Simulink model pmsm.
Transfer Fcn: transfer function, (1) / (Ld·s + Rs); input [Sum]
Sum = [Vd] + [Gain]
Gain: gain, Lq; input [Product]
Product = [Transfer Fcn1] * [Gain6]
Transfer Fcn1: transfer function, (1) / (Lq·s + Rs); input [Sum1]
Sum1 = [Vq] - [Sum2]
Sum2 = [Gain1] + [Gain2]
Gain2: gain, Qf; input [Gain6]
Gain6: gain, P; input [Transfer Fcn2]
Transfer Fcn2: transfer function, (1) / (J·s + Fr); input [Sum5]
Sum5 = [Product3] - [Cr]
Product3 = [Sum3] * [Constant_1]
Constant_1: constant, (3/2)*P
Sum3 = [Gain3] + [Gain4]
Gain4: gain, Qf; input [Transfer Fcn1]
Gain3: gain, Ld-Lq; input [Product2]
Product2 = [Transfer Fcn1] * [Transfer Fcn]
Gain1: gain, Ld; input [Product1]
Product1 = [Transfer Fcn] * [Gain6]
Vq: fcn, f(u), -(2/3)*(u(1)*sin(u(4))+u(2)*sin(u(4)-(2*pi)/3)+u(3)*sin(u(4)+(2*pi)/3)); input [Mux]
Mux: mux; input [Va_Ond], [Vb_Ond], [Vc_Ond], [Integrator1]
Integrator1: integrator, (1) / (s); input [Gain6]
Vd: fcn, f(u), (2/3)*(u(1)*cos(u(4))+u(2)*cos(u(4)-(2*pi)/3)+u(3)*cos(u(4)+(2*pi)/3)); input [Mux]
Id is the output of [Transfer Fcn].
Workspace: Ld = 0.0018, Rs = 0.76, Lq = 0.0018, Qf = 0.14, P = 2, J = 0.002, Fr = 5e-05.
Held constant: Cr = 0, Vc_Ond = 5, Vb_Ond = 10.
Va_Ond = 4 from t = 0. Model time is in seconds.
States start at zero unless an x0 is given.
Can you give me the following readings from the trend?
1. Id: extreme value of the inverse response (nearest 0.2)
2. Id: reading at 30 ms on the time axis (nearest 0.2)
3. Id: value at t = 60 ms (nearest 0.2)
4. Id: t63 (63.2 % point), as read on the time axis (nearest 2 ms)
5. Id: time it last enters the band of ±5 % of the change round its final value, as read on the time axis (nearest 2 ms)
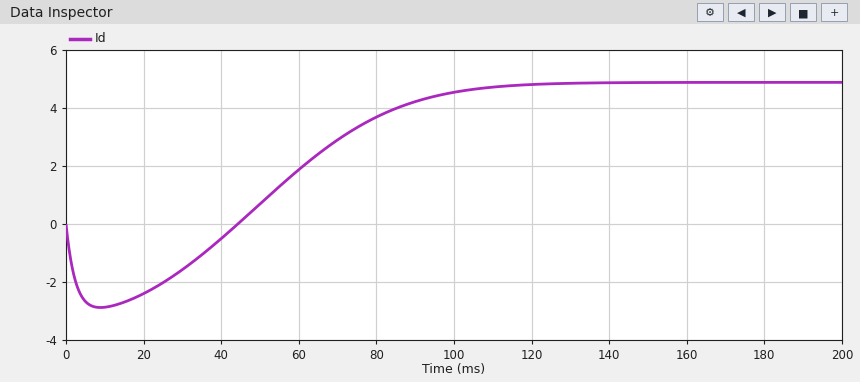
-2.8
-1.6
1.8
72 ms
104 ms
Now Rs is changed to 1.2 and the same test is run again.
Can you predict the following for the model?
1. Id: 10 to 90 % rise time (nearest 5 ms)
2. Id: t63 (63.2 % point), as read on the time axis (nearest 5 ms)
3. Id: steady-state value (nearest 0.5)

45 ms
80 ms
3.0
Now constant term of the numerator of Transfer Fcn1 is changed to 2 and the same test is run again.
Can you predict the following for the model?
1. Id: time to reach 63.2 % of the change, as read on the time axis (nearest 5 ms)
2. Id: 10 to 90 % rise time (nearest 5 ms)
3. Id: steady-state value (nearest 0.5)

65 ms
50 ms
5.0
